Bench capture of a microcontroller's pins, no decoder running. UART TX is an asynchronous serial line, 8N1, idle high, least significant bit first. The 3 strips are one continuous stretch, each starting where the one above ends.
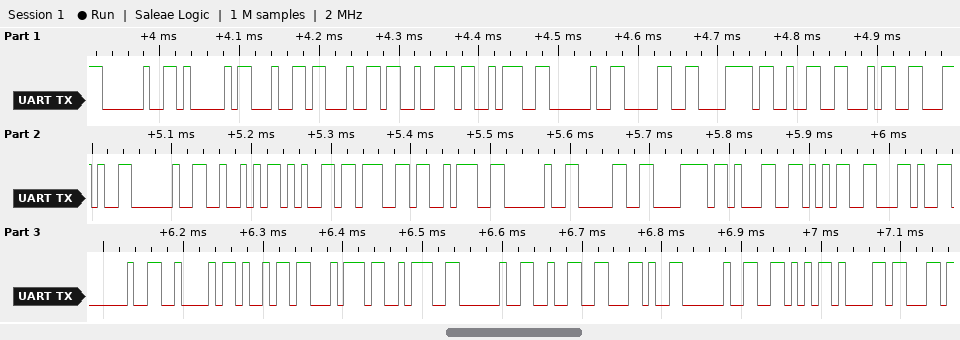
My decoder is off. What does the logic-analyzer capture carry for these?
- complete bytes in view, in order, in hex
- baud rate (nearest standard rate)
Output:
20 41 64 64 72 3A 20 30 78 32 34 2C 20 52 65 67 3A 20 30 78 31 35 2C 20 42 69 74 3A 20 32 2C 20 56 61
115200 baud
